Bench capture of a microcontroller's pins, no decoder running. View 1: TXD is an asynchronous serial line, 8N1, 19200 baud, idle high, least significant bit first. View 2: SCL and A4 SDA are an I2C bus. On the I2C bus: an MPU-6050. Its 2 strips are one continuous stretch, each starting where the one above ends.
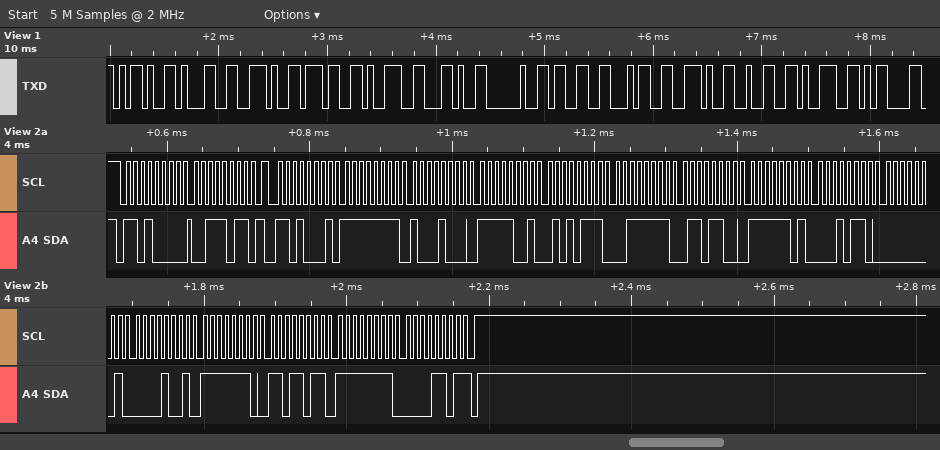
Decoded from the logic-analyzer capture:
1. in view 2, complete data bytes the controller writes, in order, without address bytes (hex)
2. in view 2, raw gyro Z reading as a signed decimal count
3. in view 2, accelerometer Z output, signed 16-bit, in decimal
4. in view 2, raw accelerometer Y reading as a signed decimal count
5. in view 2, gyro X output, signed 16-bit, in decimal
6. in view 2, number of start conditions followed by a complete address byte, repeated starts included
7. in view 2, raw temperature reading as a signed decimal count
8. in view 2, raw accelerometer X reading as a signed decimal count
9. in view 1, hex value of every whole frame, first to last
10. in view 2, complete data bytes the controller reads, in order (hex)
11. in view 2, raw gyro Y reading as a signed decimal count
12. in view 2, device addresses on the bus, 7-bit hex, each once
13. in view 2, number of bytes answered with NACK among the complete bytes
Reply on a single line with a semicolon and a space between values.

3B; -243; 16236; -1705; 265; 2; -746; -120; 2D 31 2E 37 39 2C 20 33 34 2E 32 39 0D; FF 88 F9 57 3F 6C FD 16 01 09 FE DB FF 0D; -293; 0x68; 1
